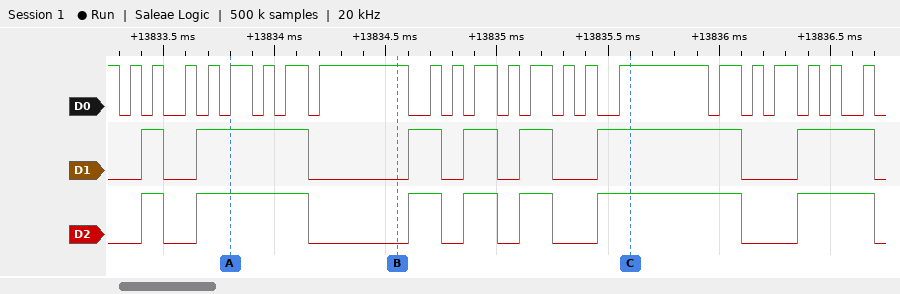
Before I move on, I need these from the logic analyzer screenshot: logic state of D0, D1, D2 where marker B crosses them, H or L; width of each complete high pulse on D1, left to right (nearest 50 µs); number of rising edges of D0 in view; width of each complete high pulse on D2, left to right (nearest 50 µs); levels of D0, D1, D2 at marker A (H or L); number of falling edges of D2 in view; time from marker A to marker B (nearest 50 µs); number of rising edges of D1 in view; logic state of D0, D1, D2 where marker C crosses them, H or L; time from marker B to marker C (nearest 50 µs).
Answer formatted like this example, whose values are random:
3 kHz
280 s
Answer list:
D0=H, D1=L, D2=L
100 µs, 500 µs, 150 µs, 150 µs, 150 µs, 650 µs, 350 µs
22
100 µs, 500 µs, 150 µs, 150 µs, 150 µs, 650 µs, 350 µs
D0=H, D1=H, D2=H
7
750 µs
7
D0=H, D1=H, D2=H
1050 µs
